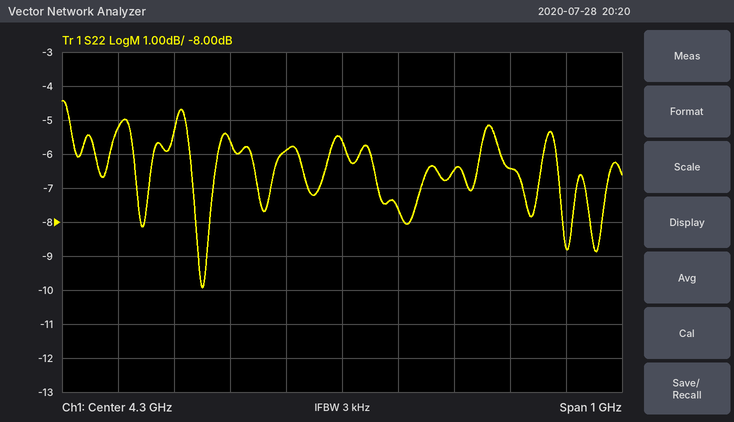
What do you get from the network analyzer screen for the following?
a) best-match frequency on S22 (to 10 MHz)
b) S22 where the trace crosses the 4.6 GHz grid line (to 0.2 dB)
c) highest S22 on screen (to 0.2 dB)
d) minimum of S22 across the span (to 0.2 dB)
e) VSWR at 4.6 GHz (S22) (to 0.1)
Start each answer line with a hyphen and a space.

- 4.05 GHz
- -6.4 dB
- -4.4 dB
- -10.0 dB
- 2.8
